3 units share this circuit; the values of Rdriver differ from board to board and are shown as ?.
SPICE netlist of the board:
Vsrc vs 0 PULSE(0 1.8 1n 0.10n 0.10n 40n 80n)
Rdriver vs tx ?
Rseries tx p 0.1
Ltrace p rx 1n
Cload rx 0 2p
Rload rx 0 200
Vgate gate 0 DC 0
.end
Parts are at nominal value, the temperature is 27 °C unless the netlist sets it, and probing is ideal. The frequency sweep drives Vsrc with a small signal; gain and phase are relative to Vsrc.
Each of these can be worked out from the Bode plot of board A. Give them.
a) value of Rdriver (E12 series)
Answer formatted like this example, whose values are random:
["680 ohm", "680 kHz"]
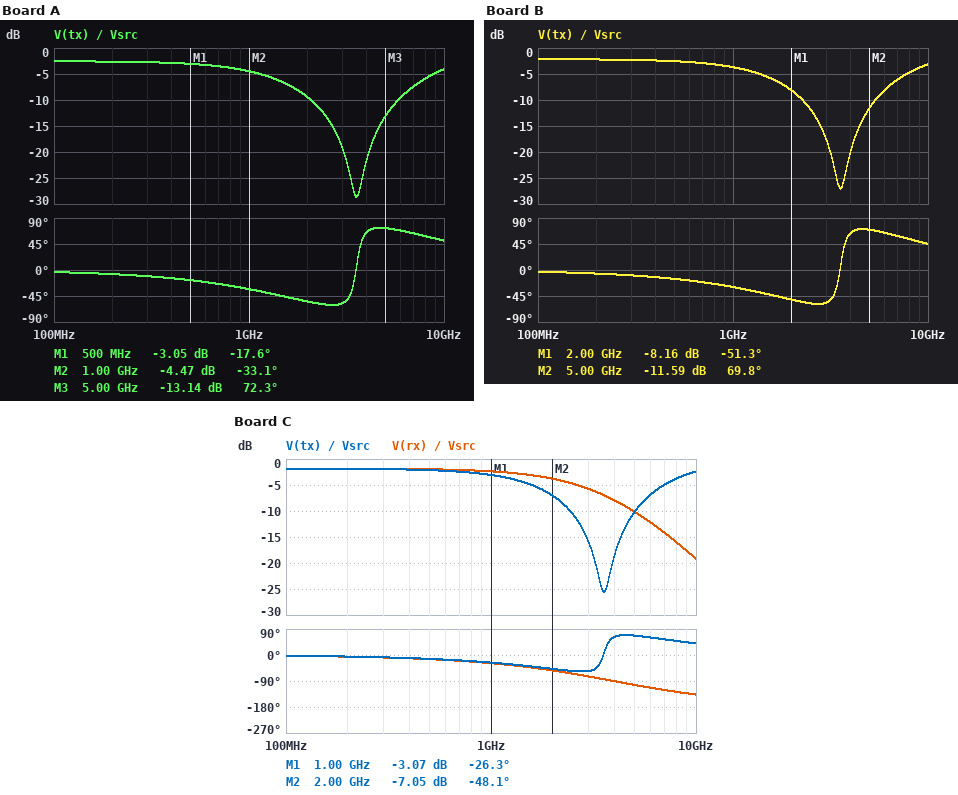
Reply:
["68 Ω"]
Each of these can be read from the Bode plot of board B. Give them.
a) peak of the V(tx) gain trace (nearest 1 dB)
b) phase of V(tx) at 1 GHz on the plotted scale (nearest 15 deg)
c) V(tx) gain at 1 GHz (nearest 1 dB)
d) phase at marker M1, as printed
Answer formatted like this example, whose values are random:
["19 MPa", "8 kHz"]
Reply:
["-2 dB", "-30 deg", "-4 dB", "-51.3 deg"]
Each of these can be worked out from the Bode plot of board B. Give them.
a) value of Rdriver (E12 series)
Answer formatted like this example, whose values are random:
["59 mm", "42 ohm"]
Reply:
["56 Ω"]
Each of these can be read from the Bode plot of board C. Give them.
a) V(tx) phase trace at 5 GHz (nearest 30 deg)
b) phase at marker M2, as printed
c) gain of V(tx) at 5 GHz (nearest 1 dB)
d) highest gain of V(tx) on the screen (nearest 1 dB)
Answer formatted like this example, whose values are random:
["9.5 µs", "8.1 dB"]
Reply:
["60 deg", "-48.1 deg", "-10 dB", "-2 dB"]
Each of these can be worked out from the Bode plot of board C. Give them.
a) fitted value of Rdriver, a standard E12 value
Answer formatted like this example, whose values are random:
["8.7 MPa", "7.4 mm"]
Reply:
["47 Ω"]
